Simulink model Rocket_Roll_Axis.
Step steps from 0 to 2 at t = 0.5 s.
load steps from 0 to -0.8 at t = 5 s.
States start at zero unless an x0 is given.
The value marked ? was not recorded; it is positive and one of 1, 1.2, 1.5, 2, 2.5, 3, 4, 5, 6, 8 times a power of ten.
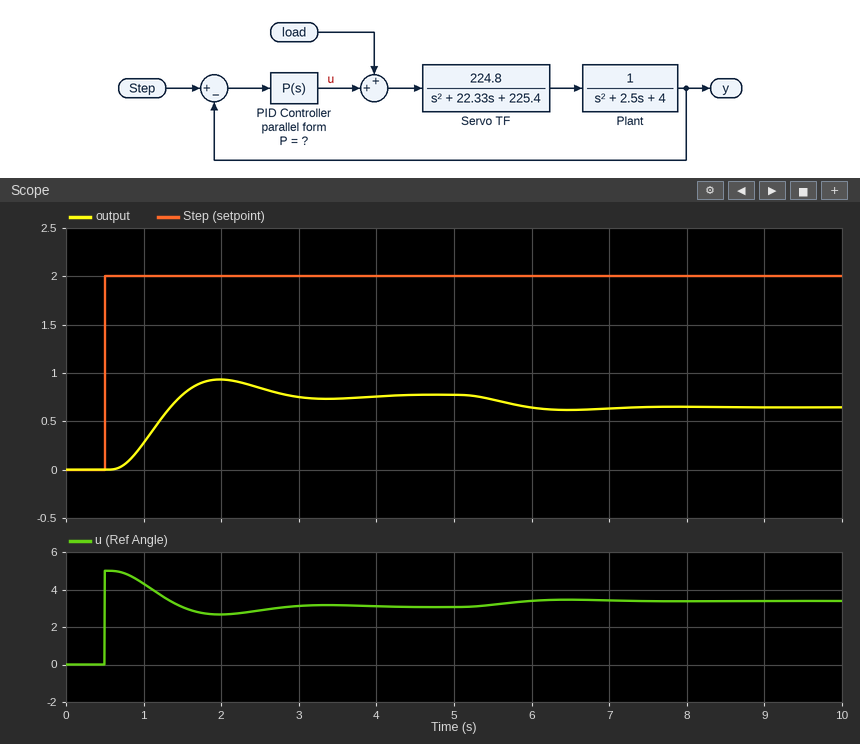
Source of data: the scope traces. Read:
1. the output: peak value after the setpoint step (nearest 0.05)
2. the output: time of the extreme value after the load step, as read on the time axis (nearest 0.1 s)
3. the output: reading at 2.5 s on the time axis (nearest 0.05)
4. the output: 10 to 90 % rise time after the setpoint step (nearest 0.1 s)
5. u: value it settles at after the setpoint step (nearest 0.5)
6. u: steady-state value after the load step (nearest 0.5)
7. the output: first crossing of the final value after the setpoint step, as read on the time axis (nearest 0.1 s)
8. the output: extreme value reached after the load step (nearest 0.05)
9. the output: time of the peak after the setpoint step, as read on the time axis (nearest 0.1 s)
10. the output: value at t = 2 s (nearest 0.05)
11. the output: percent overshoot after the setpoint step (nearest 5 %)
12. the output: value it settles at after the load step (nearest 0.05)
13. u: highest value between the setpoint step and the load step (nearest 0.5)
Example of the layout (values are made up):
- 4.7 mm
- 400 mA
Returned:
- 0.95
- 6.5 s
- 0.85
- 0.6 s
- 3.0
- 3.5
- 1.5 s
- 0.60
- 2.0 s
- 0.95
- 20 %
- 0.65
- 5.0
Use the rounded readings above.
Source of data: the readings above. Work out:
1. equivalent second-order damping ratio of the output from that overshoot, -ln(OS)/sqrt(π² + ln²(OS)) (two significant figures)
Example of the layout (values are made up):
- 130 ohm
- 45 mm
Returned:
- 0.46
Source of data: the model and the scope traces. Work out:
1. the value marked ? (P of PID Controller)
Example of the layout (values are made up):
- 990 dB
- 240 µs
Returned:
- 2.5
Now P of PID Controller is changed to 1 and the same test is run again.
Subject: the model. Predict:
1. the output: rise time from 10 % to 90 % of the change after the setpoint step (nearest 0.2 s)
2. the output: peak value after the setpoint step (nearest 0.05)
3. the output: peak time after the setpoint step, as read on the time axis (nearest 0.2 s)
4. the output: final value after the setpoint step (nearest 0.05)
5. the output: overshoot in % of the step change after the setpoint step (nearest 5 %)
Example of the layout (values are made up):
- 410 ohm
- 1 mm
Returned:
- 0.8 s
- 0.45
- 2.2 s
- 0.40
- 15 %
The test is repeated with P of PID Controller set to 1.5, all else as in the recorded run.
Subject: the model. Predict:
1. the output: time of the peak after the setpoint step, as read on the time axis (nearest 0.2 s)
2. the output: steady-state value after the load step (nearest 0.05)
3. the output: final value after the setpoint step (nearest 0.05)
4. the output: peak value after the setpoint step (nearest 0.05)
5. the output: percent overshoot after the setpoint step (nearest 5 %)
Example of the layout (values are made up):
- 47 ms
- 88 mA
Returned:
- 2.2 s
- 0.40
- 0.55
- 0.65
- 15 %
